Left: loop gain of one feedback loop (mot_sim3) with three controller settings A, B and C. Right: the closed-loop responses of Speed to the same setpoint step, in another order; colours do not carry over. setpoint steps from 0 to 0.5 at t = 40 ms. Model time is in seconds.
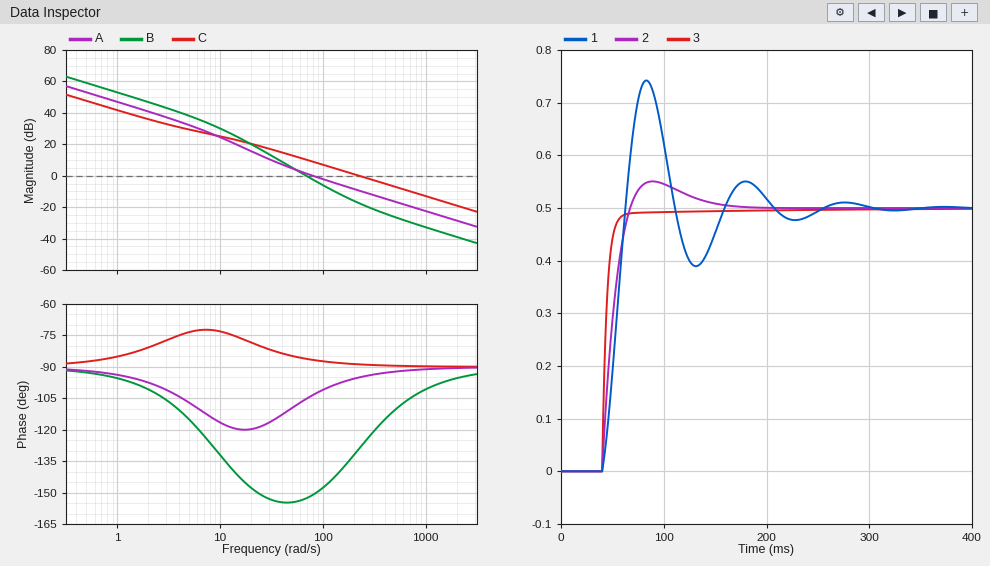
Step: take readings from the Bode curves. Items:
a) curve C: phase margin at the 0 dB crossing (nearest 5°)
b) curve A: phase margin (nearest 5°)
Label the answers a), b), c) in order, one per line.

a) 90°
b) 75°
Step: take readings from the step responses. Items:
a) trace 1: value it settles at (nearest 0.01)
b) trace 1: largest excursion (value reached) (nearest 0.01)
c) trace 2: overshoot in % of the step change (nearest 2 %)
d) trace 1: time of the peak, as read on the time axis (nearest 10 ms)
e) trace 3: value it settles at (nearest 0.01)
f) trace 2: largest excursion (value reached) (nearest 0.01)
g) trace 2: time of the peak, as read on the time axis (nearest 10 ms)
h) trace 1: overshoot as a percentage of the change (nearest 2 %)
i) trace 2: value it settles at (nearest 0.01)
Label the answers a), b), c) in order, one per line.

a) 0.50
b) 0.74
c) 10 %
d) 80 ms
e) 0.50
f) 0.55
g) 90 ms
h) 48 %
i) 0.50
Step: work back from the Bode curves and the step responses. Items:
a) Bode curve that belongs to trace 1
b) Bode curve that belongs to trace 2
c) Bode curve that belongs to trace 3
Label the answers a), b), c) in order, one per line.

a) B
b) A
c) C
